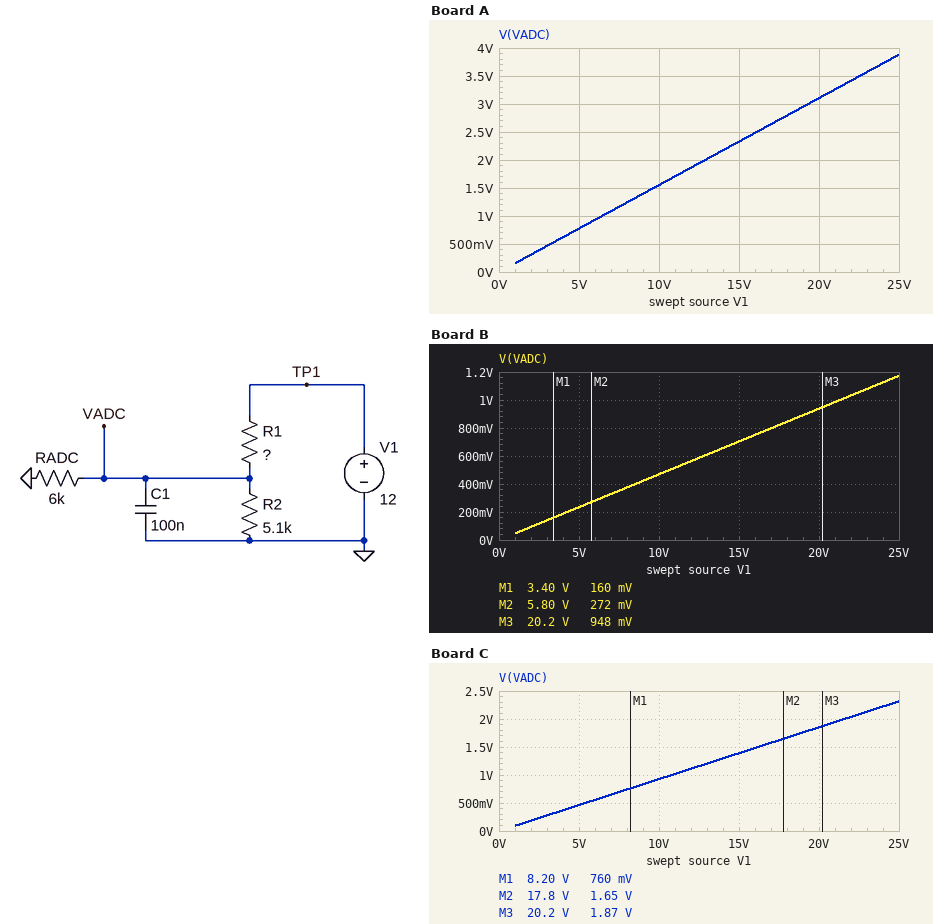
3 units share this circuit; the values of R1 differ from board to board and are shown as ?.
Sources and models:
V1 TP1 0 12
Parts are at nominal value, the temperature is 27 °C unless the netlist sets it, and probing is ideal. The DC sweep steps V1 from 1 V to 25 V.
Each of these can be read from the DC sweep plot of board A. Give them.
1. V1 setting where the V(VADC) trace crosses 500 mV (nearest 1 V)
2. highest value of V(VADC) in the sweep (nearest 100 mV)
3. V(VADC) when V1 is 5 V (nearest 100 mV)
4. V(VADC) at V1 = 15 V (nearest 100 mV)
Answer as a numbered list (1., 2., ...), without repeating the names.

1. 3 V
2. 3.9 V
3. 800 mV
4. 2.3 V
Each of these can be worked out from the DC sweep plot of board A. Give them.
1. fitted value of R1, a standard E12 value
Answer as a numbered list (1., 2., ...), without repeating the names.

1. 15 kΩ
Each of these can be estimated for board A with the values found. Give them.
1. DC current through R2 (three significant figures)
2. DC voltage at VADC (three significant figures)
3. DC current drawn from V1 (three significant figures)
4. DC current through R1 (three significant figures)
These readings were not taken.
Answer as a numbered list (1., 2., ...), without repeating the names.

1. 365 µA
2. 1.86 V
3. 676 µA
4. 676 µA
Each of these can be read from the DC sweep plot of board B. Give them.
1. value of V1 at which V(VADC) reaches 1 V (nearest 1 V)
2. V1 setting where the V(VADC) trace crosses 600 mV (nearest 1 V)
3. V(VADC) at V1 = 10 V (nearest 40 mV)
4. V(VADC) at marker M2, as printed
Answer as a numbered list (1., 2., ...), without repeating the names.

1. 21 V
2. 13 V
3. 480 mV
4. 272 mV
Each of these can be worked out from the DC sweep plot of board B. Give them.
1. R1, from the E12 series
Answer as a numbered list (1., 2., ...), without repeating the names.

1. 56 kΩ
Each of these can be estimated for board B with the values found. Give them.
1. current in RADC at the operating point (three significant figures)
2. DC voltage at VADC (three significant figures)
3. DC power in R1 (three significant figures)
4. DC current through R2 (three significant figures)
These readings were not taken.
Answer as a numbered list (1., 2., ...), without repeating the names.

1. 93.8 µA
2. 563 mV
3. 2.34 mW
4. 110 µA
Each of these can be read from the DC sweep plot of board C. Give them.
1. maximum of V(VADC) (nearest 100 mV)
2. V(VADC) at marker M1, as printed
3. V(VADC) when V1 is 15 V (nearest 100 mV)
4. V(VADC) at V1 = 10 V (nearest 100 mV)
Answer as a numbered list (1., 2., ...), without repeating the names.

1. 2.3 V
2. 760 mV
3. 1.4 V
4. 900 mV
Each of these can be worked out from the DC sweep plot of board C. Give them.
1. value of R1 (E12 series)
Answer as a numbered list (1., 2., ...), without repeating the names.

1. 27 kΩ
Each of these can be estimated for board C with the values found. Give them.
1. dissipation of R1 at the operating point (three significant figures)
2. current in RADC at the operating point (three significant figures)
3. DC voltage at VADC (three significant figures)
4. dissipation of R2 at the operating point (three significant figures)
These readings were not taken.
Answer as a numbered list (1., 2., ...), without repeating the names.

1. 4.39 mW
2. 185 µA
3. 1.11 V
4. 242 µW
